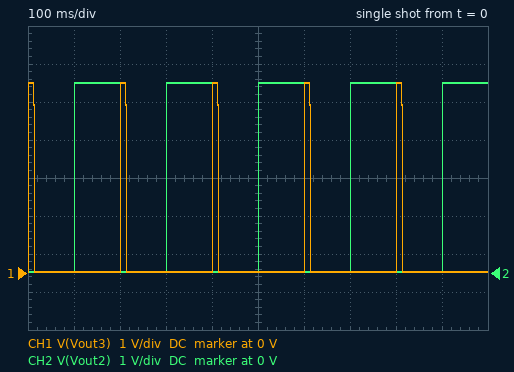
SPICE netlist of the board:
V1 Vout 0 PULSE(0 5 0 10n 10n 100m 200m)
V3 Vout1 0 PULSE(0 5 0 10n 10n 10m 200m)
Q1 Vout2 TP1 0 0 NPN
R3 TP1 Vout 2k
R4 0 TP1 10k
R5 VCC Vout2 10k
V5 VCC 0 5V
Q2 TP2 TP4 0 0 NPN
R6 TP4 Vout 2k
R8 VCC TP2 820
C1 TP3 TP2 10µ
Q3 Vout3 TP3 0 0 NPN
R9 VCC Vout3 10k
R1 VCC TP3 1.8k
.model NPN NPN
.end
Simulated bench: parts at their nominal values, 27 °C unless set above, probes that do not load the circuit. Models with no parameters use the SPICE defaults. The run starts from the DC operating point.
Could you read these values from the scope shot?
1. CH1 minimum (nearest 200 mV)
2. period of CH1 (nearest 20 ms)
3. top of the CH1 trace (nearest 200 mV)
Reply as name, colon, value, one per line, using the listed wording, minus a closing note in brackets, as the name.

CH1 minimum: 0 V
period of CH1: 200 ms
top of the CH1 trace: 5.0 V
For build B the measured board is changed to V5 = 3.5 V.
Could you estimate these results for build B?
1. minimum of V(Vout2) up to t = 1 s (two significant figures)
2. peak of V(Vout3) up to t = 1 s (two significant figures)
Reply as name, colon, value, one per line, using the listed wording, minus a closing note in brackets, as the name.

minimum of V(Vout2) up to t = 1 s: 20 mV
peak of V(Vout3) up to t = 1 s: 3.5 V
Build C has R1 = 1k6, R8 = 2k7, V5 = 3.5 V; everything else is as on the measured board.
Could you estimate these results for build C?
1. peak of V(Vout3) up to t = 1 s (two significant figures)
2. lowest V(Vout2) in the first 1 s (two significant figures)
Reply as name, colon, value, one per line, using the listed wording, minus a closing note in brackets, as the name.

peak of V(Vout3) up to t = 1 s: 3.5 V
lowest V(Vout2) in the first 1 s: 20 mV
